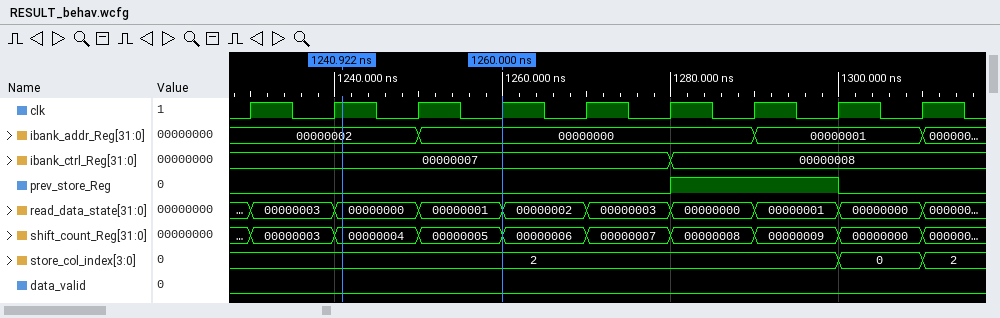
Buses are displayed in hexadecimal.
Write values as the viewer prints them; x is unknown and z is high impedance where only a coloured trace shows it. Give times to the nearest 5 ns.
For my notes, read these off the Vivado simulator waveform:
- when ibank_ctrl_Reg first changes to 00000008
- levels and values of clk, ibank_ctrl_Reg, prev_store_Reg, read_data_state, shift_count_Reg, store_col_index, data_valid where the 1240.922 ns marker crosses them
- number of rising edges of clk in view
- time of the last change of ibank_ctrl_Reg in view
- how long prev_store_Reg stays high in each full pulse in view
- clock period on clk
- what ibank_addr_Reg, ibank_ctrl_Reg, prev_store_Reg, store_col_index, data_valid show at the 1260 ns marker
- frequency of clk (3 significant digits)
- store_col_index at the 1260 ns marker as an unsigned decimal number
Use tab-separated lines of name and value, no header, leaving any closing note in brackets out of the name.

when ibank_ctrl_Reg first changes to 00000008	1280 ns
levels and values of clk, ibank_ctrl_Reg, prev_store_Reg, read_data_state, shift_count_Reg, store_col_index, data_valid where the 1240.922 ns marker crosses them	clk=1, ibank_ctrl_Reg=00000007, prev_store_Reg=0, read_data_state=00000000, shift_count_Reg=00000004, store_col_index=2, data_valid=0
number of rising edges of clk in view	9
time of the last change of ibank_ctrl_Reg in view	1280 ns
how long prev_store_Reg stays high in each full pulse in view	20 ns
clock period on clk	10 ns
what ibank_addr_Reg, ibank_ctrl_Reg, prev_store_Reg, store_col_index, data_valid show at the 1260 ns marker	ibank_addr_Reg=00000000, ibank_ctrl_Reg=00000007, prev_store_Reg=0, store_col_index=2, data_valid=0
frequency of clk	100 MHz
store_col_index at the 1260 ns marker as an unsigned decimal number	2
